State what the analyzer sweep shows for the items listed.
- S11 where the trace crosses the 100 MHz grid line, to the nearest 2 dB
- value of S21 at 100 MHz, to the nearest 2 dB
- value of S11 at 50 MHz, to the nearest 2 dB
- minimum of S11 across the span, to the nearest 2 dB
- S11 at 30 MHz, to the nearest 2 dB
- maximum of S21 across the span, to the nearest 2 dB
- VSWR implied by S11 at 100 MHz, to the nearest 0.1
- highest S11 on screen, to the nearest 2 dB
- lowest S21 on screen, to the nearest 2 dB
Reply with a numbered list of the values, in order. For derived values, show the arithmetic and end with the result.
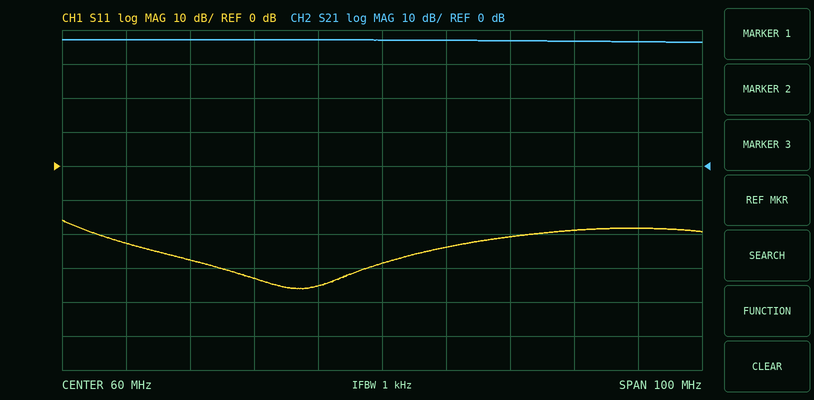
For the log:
1. -18 dB
2. 36 dB
3. -36 dB
4. -36 dB
5. -28 dB
6. 38 dB
7. |Γ| = 10^(-18/20) = 0.1259; VSWR = (1 + 0.1259)/(1 − 0.1259) ≈ 1.3
8. -16 dB
9. 36 dB
